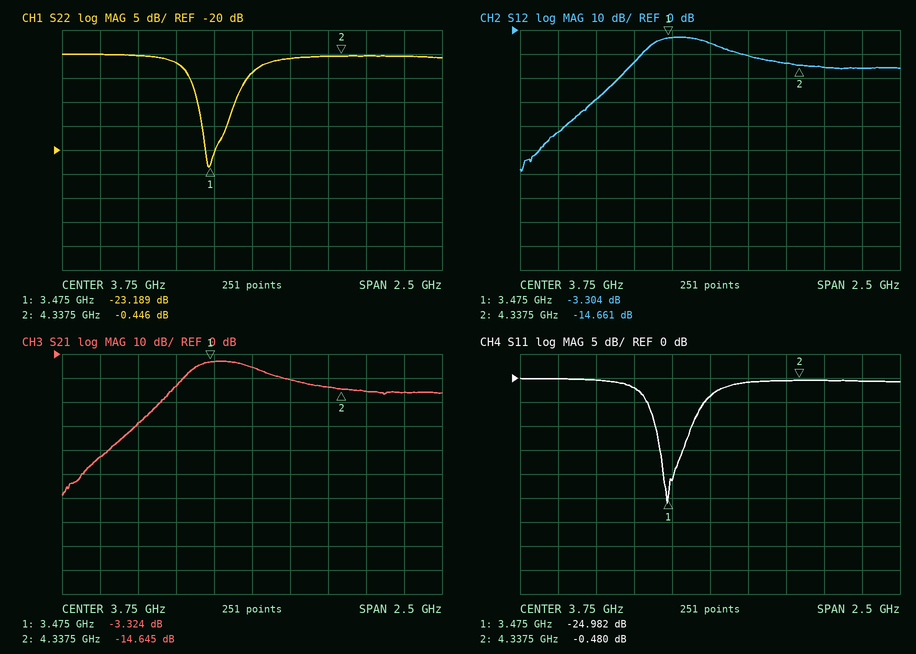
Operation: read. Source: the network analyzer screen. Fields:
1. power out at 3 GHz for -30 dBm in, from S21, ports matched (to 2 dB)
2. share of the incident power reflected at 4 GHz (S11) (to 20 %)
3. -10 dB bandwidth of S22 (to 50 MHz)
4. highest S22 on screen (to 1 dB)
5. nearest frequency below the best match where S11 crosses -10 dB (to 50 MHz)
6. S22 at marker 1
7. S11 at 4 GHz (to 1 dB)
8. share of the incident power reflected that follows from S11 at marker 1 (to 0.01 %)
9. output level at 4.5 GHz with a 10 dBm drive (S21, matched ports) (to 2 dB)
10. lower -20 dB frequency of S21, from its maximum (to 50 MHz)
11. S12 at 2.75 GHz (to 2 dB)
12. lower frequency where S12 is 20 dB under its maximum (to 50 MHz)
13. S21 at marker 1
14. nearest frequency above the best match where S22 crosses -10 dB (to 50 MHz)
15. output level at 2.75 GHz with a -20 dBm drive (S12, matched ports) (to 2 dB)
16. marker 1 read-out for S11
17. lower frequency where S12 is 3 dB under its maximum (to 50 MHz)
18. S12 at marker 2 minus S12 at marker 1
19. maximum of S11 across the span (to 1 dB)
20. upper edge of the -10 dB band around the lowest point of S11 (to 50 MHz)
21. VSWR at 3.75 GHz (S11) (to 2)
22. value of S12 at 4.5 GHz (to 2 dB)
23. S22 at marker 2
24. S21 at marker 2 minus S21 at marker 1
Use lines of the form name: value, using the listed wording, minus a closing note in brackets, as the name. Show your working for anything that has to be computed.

power out at 3 GHz for -30 dBm in, from S21, ports matched: -30 dBm + (-28 dB) = -58 dBm
share of the incident power reflected at 4 GHz (S11): 10^(-1/10) ≈ 79.4 %, so 80 % to the nearest 20 %
-10 dB bandwidth of S22: 3.65 GHz − 3.40 GHz = 250 MHz
highest S22 on screen: 0 dB
nearest frequency below the best match where S11 crosses -10 dB: 3.40 GHz
S22 at marker 1: -23.189 dB
S11 at 4 GHz: -1 dB
share of the incident power reflected that follows from S11 at marker 1: 10^(-24.982/10) ≈ 0.32 %
output level at 4.5 GHz with a 10 dBm drive (S21, matched ports): 10 dBm + (-16 dB) = -6 dBm
lower -20 dB frequency of S21, from its maximum: 3.10 GHz
S12 at 2.75 GHz: -42 dB
lower frequency where S12 is 20 dB under its maximum: 3.10 GHz
S21 at marker 1: -3.324 dB
nearest frequency above the best match where S22 crosses -10 dB: 3.65 GHz
output level at 2.75 GHz with a -20 dBm drive (S12, matched ports): -20 dBm + (-42 dB) = -62 dBm
marker 1 read-out for S11: -24.982 dB
lower frequency where S12 is 3 dB under its maximum: 3.35 GHz
S12 at marker 2 minus S12 at marker 1: -14.661 − (-3.304) = -11.357 dB
maximum of S11 across the span: 0 dB
upper edge of the -10 dB band around the lowest point of S11: 3.65 GHz
VSWR at 3.75 GHz (S11): |Γ| = 10^(-4/20) = 0.6310; VSWR = (1 + 0.6310)/(1 − 0.6310) ≈ 4
value of S12 at 4.5 GHz: -16 dB
S22 at marker 2: -0.446 dB
S21 at marker 2 minus S21 at marker 1: -14.645 − (-3.324) = -11.321 dB
